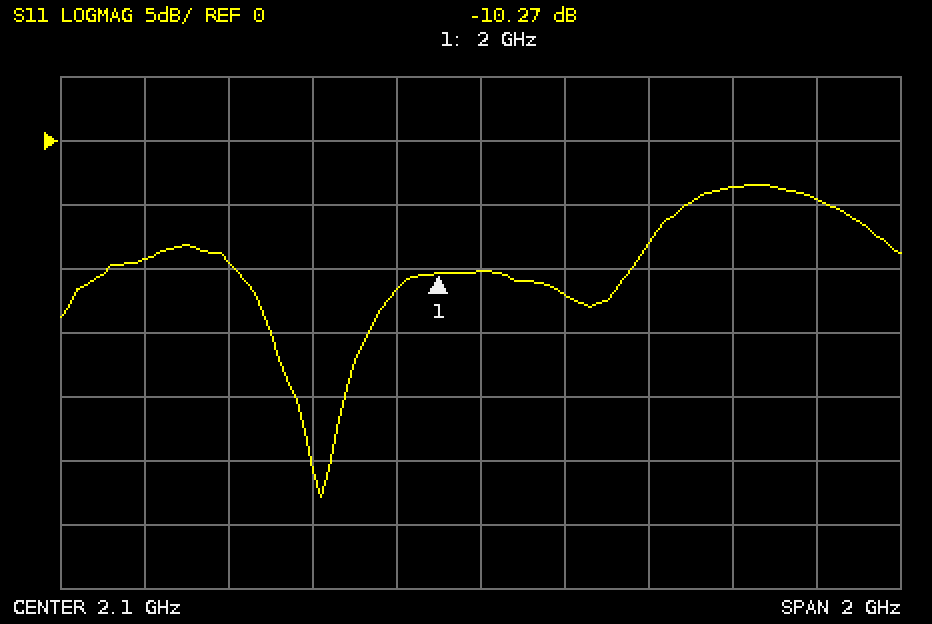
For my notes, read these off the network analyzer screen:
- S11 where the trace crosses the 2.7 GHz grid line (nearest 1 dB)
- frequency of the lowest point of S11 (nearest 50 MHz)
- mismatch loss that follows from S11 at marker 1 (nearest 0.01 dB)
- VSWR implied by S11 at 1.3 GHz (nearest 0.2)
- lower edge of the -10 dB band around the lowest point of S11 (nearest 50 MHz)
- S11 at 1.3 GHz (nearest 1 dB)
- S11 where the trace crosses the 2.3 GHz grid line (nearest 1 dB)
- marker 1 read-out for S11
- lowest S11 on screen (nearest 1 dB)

-4 dB
1.70 GHz
0.43 dB
2.0
1.50 GHz
-9 dB
-12 dB
-10.27 dB
-28 dB
